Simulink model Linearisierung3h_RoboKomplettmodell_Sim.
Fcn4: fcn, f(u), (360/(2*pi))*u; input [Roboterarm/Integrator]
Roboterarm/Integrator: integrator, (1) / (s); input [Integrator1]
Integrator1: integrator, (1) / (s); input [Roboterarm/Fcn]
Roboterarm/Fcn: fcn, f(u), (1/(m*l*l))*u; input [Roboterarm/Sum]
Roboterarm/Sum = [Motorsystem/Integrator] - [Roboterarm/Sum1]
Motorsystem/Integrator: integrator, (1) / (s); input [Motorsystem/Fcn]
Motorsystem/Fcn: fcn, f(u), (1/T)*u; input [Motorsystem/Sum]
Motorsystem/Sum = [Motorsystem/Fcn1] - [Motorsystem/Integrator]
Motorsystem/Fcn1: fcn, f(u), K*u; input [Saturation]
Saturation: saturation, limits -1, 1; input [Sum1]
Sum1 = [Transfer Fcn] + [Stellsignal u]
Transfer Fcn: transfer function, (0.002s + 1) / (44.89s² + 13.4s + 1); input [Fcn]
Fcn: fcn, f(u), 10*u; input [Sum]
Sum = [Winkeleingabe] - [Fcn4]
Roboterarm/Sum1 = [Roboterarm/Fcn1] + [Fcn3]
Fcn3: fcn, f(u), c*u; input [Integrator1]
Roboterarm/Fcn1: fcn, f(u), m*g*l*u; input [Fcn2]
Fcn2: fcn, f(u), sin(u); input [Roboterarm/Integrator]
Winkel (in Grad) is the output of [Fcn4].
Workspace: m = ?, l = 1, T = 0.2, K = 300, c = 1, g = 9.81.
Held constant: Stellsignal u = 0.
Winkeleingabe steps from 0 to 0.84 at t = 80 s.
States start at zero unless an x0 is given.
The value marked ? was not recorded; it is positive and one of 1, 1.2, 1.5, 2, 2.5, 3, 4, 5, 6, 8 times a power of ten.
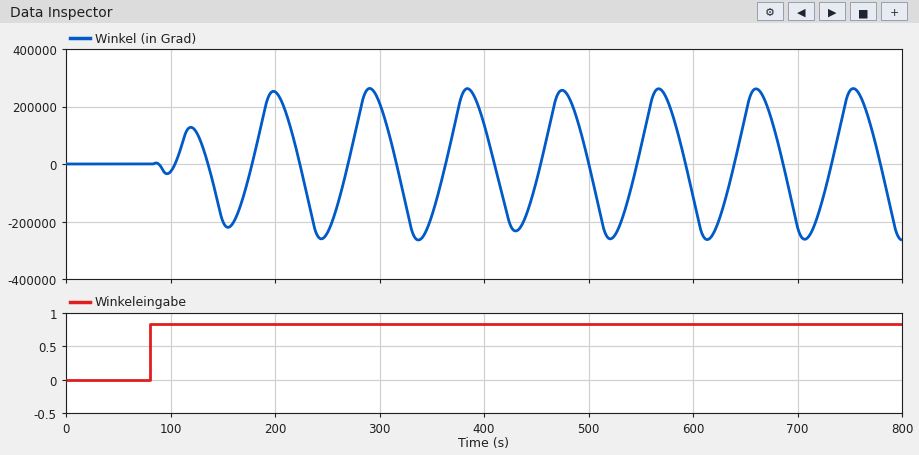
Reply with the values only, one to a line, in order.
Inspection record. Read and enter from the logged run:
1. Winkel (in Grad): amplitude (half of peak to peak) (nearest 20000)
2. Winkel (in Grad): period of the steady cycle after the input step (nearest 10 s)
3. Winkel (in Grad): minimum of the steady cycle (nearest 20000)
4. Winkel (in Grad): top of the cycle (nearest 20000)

260000
90 s
-260000
260000
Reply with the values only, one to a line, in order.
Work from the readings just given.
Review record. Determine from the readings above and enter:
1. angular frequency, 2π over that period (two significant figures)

0.070 rad/s
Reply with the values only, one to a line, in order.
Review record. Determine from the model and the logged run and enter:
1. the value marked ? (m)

12
